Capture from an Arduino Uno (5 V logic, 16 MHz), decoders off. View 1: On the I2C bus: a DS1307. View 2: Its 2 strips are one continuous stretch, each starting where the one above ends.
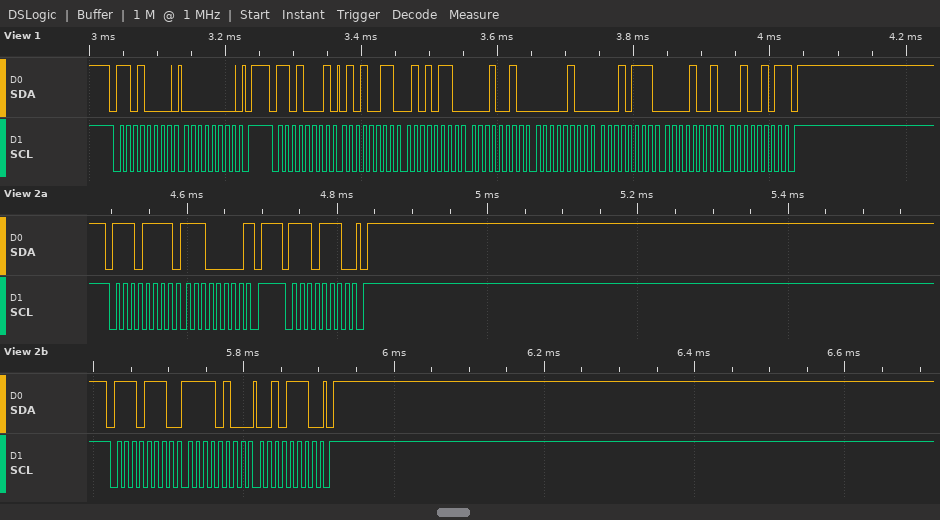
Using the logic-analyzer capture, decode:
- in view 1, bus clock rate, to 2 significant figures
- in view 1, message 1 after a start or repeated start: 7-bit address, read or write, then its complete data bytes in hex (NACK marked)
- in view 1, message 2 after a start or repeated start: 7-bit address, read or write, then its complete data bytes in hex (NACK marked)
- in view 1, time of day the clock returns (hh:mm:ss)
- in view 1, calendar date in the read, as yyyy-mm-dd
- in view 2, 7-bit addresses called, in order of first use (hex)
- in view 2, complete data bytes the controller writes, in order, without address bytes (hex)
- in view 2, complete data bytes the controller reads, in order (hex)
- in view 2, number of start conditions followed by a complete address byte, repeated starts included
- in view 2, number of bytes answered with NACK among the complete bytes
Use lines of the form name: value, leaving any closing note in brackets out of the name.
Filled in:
in view 1, bus clock rate, to 2 significant figures: 100 kHz
in view 1, message 1 after a start or repeated start: 7-bit address, read or write, then its complete data bytes in hex: 0x68 write: 00
in view 1, message 2 after a start or repeated start: 7-bit address, read or write, then its complete data bytes in hex: 0x68 read: 53 56 12 04 17 09 25 NACK
in view 1, time of day the clock returns: 12:56:53
in view 1, calendar date in the read, as yyyy-mm-dd: 2025-09-17
in view 2, 7-bit addresses called, in order of first use: 0x77
in view 2, complete data bytes the controller writes, in order, without address bytes: F4 2E
in view 2, complete data bytes the controller reads, in order: E0
in view 2, number of start conditions followed by a complete address byte, repeated starts included: 3
in view 2, number of bytes answered with NACK among the complete bytes: 1
